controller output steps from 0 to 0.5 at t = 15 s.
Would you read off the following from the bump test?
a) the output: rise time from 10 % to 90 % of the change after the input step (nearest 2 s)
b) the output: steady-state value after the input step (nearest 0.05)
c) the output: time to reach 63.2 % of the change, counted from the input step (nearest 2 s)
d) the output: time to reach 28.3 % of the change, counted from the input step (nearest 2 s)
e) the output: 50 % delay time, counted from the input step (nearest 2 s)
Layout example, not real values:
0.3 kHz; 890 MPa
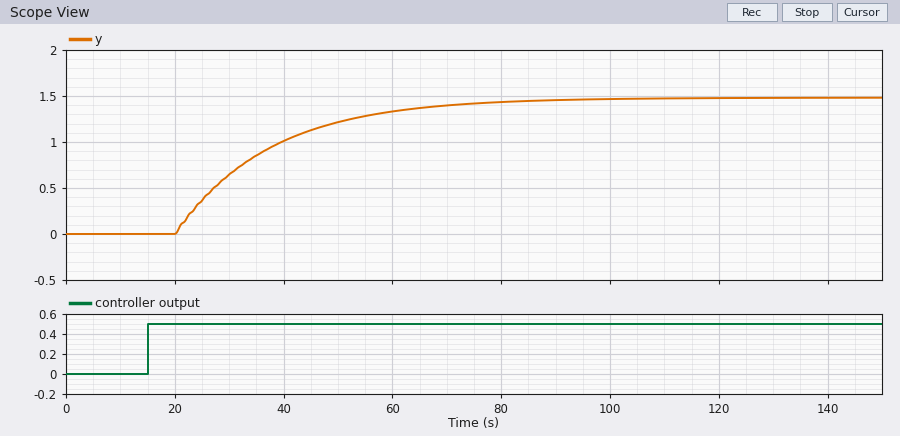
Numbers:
38 s; 1.50; 22 s; 10 s; 18 s
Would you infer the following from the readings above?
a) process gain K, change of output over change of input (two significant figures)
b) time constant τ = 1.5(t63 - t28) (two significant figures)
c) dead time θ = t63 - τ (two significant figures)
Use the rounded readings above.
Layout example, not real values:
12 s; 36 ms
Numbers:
3.0; 18 s; 4.0 s
